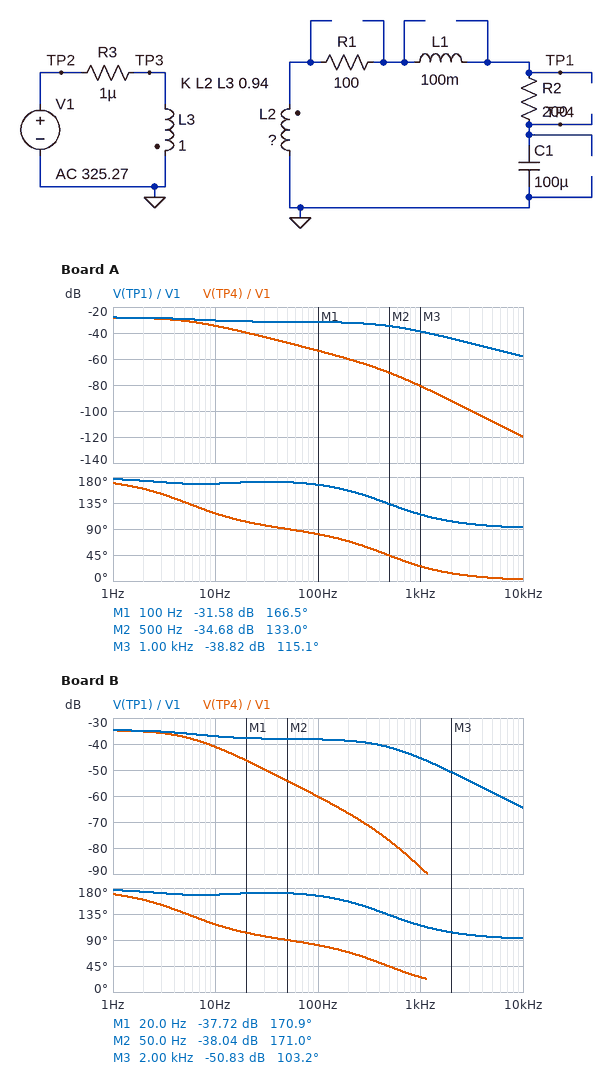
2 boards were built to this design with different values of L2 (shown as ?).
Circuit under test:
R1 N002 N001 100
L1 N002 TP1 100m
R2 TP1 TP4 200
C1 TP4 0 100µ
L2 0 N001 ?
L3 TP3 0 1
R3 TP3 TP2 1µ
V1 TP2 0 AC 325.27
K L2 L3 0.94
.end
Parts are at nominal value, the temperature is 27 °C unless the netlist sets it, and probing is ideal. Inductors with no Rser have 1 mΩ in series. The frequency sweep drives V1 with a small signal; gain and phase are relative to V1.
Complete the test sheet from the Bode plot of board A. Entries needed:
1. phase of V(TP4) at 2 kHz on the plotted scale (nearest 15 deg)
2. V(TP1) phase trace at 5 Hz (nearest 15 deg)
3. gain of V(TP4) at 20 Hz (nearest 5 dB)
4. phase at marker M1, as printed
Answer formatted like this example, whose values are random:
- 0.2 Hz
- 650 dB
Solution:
- 15 deg
- 165 deg
- -40 dB
- 166.5 deg
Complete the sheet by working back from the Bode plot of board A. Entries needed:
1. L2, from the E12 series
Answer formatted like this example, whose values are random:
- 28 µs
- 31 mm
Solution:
- 1.8 mH
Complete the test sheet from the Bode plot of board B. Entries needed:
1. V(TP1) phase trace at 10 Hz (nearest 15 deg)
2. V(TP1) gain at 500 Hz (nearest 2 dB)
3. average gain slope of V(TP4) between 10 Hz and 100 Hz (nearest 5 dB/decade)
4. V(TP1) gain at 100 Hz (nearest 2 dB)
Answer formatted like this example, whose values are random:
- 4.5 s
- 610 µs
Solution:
- 165 deg
- -42 dB
- -20 dB/decade
- -38 dB
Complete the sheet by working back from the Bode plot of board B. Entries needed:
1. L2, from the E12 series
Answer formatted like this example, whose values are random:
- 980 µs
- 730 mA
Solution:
- 390 µH
